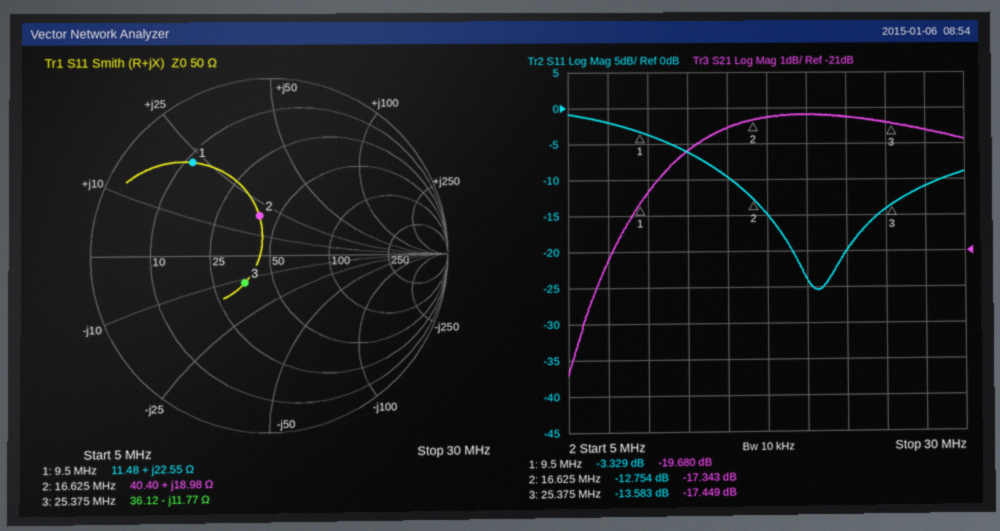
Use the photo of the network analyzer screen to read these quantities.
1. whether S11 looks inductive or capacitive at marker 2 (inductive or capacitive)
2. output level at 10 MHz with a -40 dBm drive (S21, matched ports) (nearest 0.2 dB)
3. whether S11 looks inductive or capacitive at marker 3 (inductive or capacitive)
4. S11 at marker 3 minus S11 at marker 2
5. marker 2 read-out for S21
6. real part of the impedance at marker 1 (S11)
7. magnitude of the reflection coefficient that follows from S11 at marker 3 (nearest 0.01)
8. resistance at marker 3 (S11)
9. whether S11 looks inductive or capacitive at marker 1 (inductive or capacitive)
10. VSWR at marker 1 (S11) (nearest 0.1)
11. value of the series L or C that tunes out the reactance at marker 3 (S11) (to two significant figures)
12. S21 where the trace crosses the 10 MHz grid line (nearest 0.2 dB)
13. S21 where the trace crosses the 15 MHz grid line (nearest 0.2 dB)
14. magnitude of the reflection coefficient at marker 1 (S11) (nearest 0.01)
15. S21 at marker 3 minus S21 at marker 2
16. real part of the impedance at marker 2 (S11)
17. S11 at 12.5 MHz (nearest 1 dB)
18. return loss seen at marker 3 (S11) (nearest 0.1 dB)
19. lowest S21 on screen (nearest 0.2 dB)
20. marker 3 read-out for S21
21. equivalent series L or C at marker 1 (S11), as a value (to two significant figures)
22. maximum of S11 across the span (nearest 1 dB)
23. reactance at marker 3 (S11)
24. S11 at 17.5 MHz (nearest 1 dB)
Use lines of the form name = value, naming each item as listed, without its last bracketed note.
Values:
whether S11 looks inductive or capacitive at marker 2 = inductive
output level at 10 MHz with a -40 dBm drive (S21, matched ports) = -59.4 dBm
whether S11 looks inductive or capacitive at marker 3 = capacitive
S11 at marker 3 minus S11 at marker 2 = -0.829 dB
marker 2 read-out for S21 = -17.343 dB
real part of the impedance at marker 1 = 11.48 Ω
magnitude of the reflection coefficient that follows from S11 at marker 3 = 0.21
resistance at marker 3 = 36.12 Ω
whether S11 looks inductive or capacitive at marker 1 = inductive
VSWR at marker 1 (S11) = 5.3
value of the series L or C that tunes out the reactance at marker 3 (S11) = 74 nH
S21 where the trace crosses the 10 MHz grid line = -19.4 dB
S21 where the trace crosses the 15 MHz grid line = -17.6 dB
magnitude of the reflection coefficient at marker 1 (S11) = 0.68
S21 at marker 3 minus S21 at marker 2 = -0.106 dB
real part of the impedance at marker 2 = 40.40 Ω
S11 at 12.5 MHz = -6 dB
return loss seen at marker 3 (S11) = 13.6 dB
lowest S21 on screen = -24.4 dB
marker 3 read-out for S21 = -17.449 dB
equivalent series L or C at marker 1 (S11), as a value = 380 nH
maximum of S11 across the span = -1 dB
reactance at marker 3 = -11.77 Ω
S11 at 17.5 MHz = -15 dB
